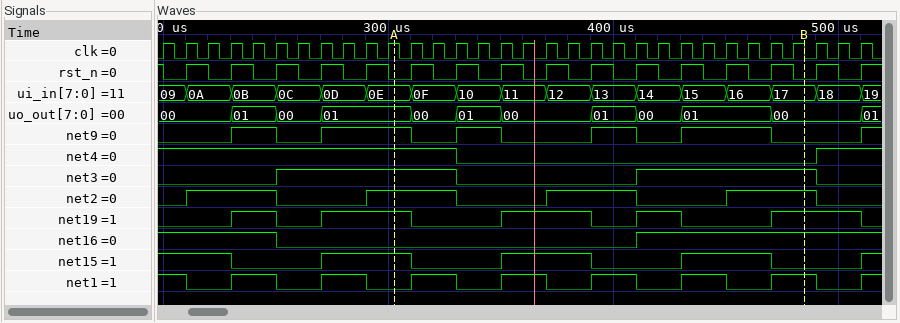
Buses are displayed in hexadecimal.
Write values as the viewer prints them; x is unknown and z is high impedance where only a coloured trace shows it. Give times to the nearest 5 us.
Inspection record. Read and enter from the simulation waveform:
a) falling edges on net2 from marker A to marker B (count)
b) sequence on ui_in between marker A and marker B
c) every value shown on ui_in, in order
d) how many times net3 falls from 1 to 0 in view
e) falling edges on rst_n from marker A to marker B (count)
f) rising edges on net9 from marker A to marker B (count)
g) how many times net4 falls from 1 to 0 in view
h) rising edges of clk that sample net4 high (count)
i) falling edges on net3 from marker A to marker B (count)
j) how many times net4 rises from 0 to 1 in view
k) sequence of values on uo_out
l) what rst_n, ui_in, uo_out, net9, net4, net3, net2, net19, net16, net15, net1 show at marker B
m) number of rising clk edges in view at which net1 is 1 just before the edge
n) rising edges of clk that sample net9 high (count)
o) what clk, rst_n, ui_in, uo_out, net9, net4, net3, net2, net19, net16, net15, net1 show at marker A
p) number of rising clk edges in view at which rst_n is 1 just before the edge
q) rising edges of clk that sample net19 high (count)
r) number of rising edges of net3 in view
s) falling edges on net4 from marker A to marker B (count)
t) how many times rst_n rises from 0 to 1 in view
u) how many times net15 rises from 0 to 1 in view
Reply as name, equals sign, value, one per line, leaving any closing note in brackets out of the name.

falling edges on net2 from marker A to marker B = 2
sequence on ui_in between marker A and marker B = 0E, 0F, 10, 11, 12, 13, 14, 15, 16, 17
every value shown on ui_in, in order = 09, 0A, 0B, 0C, 0D, 0E, 0F, 10, 11, 12, 13, 14, 15, 16, 17, 18, 19
how many times net3 falls from 1 to 0 in view = 2
falling edges on rst_n from marker A to marker B = 9
rising edges on net9 from marker A to marker B = 3
how many times net4 falls from 1 to 0 in view = 1
rising edges of clk that sample net4 high = 16
falling edges on net3 from marker A to marker B = 1
how many times net4 rises from 0 to 1 in view = 1
sequence of values on uo_out = 00, 01, 00, 01, 00, 01, 00, 01, 00, 01, 00, 01
what rst_n, ui_in, uo_out, net9, net4, net3, net2, net19, net16, net15, net1 show at marker B = rst_n=0, ui_in=17, uo_out=00, net9=0, net4=0, net3=1, net2=1, net19=1, net16=1, net15=0, net1=1
number of rising clk edges in view at which net1 is 1 just before the edge = 16
rising edges of clk that sample net9 high = 14
what clk, rst_n, ui_in, uo_out, net9, net4, net3, net2, net19, net16, net15, net1 show at marker A = clk=1, rst_n=0, ui_in=0E, uo_out=01, net9=1, net4=1, net3=1, net2=1, net19=1, net16=0, net15=1, net1=0
number of rising clk edges in view at which rst_n is 1 just before the edge = 16
rising edges of clk that sample net19 high = 16
number of rising edges of net3 in view = 2
falling edges on net4 from marker A to marker B = 1
how many times rst_n rises from 0 to 1 in view = 16
how many times net15 rises from 0 to 1 in view = 4
